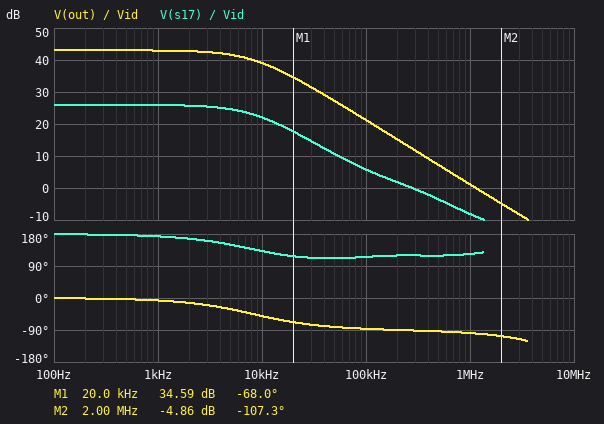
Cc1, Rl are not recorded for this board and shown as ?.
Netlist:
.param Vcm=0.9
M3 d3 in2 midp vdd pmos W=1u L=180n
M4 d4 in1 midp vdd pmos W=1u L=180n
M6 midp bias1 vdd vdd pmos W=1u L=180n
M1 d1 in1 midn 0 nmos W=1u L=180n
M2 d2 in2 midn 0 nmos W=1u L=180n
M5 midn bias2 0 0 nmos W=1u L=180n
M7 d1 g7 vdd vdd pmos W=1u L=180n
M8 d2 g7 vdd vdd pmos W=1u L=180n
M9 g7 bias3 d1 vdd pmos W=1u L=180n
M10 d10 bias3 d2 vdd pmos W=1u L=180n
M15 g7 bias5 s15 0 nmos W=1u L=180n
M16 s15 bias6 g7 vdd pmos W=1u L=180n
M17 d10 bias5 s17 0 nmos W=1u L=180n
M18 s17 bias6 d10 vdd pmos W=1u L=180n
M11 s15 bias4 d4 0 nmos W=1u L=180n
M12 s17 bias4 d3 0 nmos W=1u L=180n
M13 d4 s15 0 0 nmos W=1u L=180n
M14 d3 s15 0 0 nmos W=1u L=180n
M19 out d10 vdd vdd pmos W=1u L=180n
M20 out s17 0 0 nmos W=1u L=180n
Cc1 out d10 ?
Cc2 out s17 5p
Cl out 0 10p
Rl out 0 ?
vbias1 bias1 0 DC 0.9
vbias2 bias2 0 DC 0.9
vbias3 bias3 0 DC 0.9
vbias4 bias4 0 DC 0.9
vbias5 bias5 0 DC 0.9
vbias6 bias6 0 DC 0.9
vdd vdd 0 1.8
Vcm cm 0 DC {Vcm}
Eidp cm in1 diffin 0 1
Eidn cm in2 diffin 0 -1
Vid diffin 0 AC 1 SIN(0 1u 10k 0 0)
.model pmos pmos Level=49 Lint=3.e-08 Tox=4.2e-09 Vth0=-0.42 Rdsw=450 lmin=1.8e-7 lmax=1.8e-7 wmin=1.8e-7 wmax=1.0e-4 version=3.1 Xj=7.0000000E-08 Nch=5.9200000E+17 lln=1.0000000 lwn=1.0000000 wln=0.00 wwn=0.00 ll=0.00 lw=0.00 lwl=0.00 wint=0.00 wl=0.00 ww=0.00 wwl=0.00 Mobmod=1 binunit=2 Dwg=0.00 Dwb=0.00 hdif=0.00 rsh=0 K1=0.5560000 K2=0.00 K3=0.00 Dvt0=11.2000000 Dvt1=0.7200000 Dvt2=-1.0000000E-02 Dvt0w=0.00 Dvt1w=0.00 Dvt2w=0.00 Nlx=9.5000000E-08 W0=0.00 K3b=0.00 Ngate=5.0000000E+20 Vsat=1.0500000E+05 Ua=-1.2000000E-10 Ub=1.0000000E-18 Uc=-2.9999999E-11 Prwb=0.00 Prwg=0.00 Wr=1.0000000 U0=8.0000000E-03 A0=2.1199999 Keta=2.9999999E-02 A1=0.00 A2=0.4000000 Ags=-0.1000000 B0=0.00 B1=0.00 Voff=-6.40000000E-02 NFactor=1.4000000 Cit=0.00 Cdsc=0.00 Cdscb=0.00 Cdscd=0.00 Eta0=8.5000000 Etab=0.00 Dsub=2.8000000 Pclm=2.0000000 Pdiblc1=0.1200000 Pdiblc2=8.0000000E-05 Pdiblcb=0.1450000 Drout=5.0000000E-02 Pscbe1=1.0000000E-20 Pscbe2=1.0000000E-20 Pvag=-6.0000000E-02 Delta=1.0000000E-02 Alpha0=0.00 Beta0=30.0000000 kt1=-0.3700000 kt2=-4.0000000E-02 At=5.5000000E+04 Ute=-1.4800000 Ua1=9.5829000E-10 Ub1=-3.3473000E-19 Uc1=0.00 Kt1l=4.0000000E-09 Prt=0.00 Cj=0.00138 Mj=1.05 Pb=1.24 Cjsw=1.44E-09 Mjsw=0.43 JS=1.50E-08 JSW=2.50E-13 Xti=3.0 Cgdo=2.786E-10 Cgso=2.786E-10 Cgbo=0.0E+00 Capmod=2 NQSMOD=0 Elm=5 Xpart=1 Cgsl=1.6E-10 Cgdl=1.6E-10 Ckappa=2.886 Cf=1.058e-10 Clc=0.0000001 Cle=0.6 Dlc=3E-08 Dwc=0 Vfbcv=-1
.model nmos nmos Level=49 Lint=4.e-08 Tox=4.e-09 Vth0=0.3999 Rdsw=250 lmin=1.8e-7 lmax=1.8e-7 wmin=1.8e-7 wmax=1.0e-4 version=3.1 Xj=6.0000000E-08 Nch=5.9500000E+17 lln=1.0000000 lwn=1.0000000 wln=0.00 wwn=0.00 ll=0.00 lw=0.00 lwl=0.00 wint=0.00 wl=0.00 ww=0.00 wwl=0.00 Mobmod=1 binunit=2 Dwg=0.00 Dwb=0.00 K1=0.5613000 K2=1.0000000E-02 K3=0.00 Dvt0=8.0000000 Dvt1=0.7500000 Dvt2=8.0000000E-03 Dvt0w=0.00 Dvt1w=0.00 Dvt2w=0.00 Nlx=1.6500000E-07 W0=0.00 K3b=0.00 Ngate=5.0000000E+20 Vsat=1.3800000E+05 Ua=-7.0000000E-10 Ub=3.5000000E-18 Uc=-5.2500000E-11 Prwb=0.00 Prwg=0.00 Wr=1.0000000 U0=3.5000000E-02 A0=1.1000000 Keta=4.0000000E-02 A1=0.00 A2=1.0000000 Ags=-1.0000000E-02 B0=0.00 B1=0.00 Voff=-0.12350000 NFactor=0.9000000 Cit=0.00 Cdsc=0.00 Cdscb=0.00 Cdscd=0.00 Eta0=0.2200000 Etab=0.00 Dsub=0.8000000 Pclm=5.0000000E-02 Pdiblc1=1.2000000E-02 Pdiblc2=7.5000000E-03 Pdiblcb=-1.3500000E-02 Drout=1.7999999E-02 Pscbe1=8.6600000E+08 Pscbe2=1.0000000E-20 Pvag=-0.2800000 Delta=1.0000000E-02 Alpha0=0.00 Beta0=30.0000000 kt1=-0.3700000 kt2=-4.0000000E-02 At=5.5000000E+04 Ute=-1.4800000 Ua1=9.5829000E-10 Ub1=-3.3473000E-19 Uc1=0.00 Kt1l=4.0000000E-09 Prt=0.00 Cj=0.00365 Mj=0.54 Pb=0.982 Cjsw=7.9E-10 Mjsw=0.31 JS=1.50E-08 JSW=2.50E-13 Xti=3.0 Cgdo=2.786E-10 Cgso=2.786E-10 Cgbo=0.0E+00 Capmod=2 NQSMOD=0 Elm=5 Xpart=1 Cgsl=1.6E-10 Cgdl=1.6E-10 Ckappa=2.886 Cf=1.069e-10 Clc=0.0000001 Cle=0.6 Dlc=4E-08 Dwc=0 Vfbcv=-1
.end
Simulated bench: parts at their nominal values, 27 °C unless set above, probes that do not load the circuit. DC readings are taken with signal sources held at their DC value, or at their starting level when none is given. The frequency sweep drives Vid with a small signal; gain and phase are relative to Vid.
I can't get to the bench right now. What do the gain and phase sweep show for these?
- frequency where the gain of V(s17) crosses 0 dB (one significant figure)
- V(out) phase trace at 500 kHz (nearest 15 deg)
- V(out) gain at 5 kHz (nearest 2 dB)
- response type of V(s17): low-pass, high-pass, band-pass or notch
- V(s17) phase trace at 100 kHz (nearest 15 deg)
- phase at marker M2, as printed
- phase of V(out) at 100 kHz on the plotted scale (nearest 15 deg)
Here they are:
300 kHz
-90 deg
42 dB
low-pass
120 deg
-107.3 deg
-90 deg
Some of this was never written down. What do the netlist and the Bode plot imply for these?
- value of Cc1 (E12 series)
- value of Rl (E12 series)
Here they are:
2.2 pF
2.2 kΩ
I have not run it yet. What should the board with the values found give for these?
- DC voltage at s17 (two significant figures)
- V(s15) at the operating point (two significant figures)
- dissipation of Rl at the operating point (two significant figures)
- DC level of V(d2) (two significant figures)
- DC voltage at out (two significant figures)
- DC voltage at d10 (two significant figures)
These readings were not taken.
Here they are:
550 mV
550 mV
14 µW
1.2 V
180 mV
930 mV
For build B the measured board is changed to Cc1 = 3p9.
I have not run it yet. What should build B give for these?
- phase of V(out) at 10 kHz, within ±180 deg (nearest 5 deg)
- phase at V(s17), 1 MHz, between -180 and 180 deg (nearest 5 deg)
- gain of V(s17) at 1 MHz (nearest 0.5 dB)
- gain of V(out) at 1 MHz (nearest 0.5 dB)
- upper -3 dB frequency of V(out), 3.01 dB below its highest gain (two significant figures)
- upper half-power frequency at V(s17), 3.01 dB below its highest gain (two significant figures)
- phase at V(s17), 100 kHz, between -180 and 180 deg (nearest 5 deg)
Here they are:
-60 deg
115 deg
-3.0 dB
-2.0 dB
5.5 kHz
5.7 kHz
140 deg
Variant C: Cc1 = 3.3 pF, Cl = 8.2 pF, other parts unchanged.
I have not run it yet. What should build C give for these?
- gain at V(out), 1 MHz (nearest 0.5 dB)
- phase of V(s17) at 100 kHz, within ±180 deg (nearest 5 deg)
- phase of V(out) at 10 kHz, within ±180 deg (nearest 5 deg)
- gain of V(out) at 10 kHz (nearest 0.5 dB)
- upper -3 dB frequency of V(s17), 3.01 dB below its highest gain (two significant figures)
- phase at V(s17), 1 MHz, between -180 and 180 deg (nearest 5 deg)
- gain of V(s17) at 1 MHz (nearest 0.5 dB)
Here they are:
-1.0 dB
135 deg
-60 deg
37.5 dB
6.4 kHz
115 deg
-4.0 dB
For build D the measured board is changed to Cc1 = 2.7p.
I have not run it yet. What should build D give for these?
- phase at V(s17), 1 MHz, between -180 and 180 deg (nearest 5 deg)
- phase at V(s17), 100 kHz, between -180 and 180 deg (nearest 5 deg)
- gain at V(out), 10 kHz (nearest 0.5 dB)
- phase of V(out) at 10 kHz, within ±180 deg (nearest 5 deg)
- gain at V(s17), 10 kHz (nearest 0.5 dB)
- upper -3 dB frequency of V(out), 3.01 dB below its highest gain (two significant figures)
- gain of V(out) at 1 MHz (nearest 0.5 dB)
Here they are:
120 deg
130 deg
38.5 dB
-55 deg
21.5 dB
7.2 kHz
0 dB
